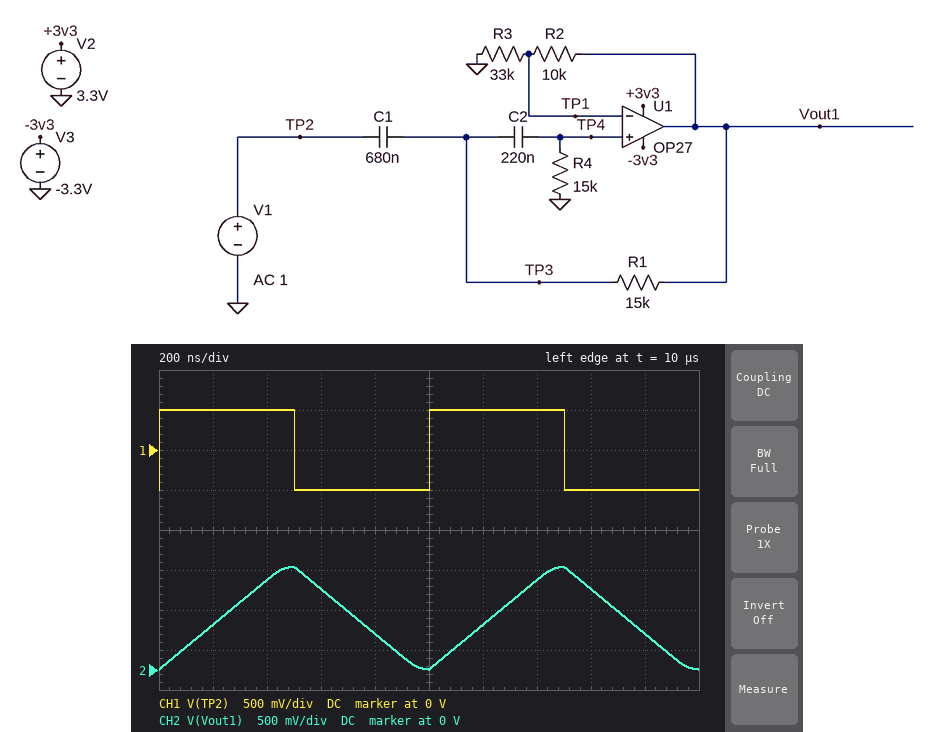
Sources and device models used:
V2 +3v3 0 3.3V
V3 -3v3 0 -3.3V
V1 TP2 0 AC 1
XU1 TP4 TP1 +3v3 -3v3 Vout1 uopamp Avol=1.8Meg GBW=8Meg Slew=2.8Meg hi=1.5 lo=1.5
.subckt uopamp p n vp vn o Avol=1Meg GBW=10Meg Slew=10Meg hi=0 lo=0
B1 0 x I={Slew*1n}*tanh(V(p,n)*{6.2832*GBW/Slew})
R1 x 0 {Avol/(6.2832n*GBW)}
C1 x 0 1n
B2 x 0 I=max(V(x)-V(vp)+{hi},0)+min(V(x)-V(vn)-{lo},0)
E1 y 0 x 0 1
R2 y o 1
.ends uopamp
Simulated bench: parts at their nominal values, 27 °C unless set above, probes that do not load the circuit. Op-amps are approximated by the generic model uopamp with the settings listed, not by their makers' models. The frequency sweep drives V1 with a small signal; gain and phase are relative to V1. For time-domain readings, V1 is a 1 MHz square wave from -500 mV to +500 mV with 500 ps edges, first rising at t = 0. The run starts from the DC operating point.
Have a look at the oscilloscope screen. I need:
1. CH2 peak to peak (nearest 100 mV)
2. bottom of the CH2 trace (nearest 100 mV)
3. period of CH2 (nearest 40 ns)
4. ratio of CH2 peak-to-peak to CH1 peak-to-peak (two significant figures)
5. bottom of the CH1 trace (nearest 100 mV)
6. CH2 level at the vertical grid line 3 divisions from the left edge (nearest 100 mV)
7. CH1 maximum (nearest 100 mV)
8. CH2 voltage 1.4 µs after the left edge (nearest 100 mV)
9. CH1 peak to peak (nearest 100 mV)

1.3 V
0 V
1.00 µs
1.3
-500 mV
1.0 V
500 mV
1.1 V
1.0 V
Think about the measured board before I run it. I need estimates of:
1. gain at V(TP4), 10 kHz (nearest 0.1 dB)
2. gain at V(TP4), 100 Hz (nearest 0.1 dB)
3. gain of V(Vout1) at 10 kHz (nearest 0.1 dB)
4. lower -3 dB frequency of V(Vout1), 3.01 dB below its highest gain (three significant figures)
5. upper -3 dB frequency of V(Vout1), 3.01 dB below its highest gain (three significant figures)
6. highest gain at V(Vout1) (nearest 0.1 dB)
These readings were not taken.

0 dB
-0.8 dB
2.3 dB
47.3 Hz
6.14 MHz
2.3 dB
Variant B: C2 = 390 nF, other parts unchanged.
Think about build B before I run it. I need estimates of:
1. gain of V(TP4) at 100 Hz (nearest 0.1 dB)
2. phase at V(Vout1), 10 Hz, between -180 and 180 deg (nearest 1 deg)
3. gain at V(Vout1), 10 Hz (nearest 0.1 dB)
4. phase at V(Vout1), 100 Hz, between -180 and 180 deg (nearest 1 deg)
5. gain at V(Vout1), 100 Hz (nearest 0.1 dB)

-0.3 dB
130 deg
-11.7 dB
22 deg
2.0 dB
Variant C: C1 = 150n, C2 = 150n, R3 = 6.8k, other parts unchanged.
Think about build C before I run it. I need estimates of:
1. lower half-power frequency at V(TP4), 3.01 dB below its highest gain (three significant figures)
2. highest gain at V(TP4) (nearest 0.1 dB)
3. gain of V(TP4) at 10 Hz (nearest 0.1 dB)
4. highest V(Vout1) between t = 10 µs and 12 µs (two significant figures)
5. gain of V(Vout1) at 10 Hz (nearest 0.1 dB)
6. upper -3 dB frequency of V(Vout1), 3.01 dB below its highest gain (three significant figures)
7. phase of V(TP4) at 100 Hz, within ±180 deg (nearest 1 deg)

60.4 Hz
5.8 dB
-33.8 dB
1.6 V
-26.0 dB
120 Hz
37 deg
